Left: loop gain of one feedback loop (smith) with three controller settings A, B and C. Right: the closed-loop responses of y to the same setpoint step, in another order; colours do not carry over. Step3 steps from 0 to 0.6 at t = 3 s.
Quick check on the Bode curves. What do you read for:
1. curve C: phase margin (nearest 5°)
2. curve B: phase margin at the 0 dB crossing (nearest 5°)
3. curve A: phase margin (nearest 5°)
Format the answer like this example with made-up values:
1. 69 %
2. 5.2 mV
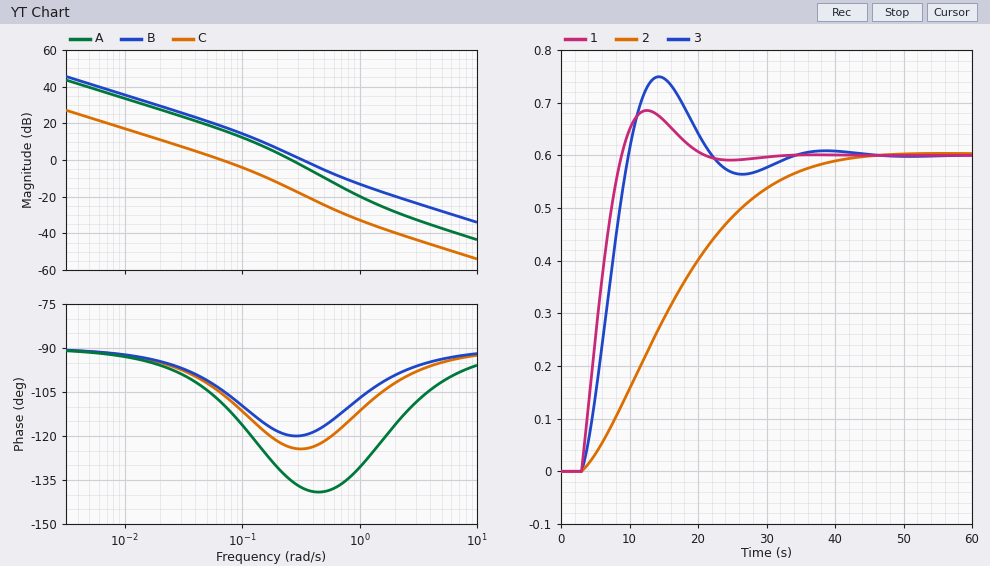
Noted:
1. 75°
2. 60°
3. 45°
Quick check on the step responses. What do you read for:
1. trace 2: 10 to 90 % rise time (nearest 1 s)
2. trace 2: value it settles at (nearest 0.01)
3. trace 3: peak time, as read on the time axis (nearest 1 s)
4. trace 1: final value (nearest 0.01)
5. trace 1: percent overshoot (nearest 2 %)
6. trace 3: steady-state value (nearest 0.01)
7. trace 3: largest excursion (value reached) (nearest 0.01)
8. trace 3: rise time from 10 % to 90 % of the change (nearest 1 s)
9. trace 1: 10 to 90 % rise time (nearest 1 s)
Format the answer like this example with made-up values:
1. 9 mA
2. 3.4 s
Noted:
1. 24 s
2. 0.60
3. 14 s
4. 0.60
5. 14 %
6. 0.60
7. 0.75
8. 5 s
9. 4 s
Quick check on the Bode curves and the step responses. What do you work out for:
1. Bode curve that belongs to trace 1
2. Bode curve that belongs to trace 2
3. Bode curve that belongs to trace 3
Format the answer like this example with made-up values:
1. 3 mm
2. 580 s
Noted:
1. B
2. C
3. A
